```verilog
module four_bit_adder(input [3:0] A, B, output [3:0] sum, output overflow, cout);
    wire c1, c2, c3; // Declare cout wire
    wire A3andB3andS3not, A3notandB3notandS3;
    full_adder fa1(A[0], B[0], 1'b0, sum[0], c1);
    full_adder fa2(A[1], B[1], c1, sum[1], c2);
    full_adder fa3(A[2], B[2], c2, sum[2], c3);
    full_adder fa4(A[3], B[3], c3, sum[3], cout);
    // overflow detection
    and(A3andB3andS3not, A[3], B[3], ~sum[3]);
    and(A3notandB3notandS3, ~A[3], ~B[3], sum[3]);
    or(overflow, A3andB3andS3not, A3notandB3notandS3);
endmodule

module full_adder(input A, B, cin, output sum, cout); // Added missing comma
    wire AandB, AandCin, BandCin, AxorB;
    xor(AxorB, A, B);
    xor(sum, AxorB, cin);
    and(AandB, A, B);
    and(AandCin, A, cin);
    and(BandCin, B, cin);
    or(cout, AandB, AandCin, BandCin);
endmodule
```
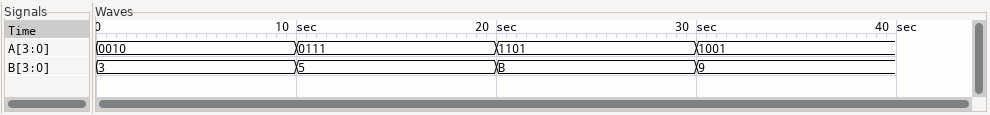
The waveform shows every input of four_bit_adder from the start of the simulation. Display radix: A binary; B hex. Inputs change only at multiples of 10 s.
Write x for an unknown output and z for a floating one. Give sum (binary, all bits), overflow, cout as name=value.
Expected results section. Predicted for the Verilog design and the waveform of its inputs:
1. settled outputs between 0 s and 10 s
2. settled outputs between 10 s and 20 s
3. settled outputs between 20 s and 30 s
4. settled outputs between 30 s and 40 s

sum=0101, overflow=0, cout=0
sum=1100, overflow=1, cout=0
sum=1000, overflow=0, cout=1
sum=0010, overflow=1, cout=1
